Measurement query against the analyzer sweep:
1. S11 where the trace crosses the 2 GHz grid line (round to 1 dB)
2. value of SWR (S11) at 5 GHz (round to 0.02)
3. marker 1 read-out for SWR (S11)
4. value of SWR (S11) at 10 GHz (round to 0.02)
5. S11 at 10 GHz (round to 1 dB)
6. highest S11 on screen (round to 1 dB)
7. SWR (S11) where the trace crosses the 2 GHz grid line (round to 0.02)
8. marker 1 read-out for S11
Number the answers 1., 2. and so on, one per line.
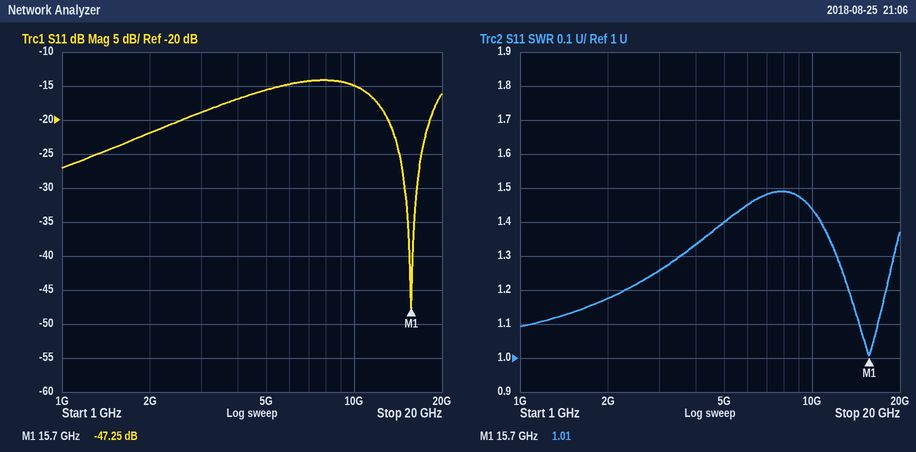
1. -22 dB
2. 1.40
3. 1.01
4. 1.44
5. -15 dB
6. -14 dB
7. 1.18
8. -47.25 dB
